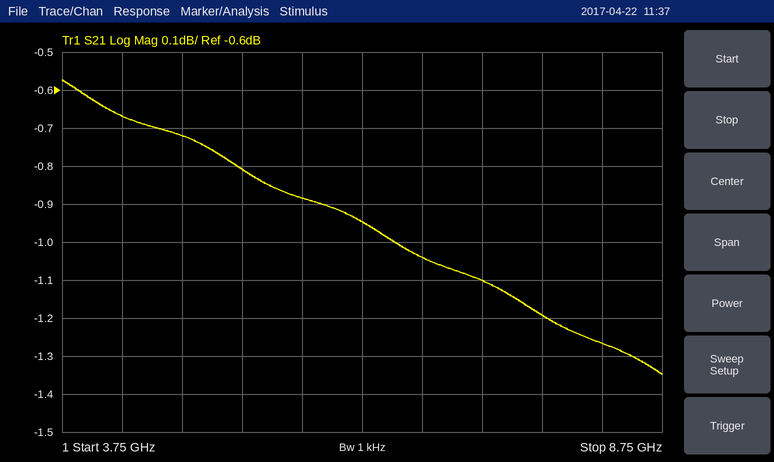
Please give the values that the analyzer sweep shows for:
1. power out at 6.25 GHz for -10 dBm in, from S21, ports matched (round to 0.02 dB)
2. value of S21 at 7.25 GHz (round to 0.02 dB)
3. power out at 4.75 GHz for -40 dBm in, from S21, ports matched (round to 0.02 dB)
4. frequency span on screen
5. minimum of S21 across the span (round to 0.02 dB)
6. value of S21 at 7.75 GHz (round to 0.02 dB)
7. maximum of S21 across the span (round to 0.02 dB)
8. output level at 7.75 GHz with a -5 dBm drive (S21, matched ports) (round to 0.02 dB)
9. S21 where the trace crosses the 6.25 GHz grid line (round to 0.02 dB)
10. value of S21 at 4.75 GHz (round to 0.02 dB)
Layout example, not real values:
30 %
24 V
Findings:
-10.94 dBm
-1.10 dB
-40.72 dBm
5 GHz
-1.34 dB
-1.20 dB
-0.58 dB
-6.20 dBm
-0.94 dB
-0.72 dB
